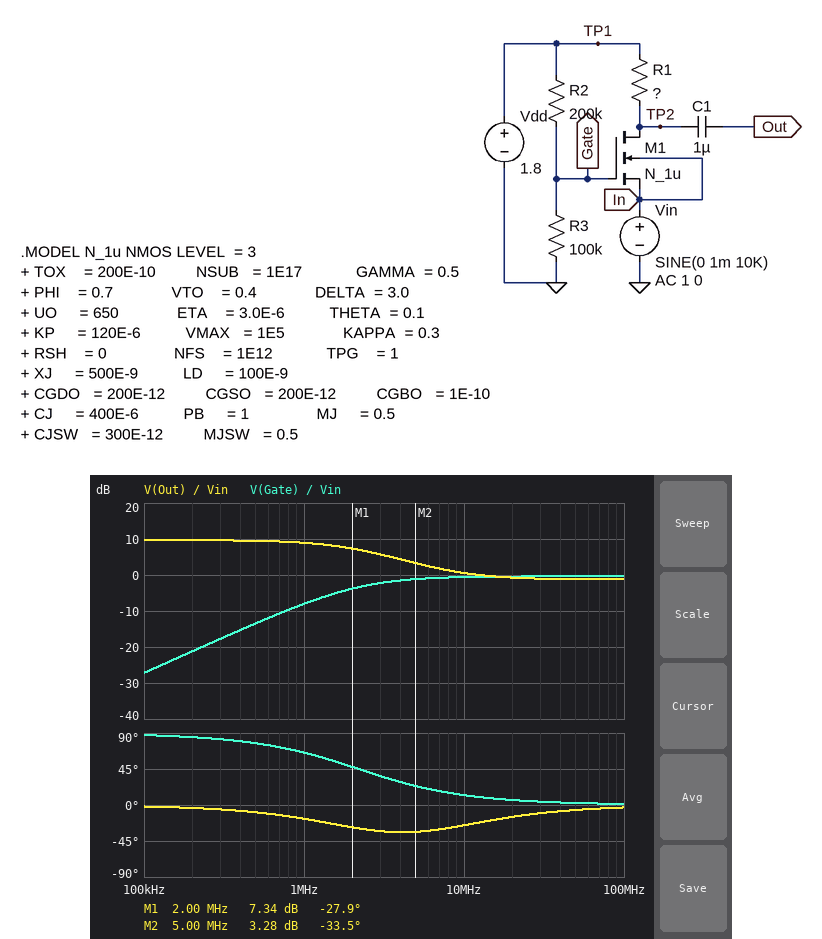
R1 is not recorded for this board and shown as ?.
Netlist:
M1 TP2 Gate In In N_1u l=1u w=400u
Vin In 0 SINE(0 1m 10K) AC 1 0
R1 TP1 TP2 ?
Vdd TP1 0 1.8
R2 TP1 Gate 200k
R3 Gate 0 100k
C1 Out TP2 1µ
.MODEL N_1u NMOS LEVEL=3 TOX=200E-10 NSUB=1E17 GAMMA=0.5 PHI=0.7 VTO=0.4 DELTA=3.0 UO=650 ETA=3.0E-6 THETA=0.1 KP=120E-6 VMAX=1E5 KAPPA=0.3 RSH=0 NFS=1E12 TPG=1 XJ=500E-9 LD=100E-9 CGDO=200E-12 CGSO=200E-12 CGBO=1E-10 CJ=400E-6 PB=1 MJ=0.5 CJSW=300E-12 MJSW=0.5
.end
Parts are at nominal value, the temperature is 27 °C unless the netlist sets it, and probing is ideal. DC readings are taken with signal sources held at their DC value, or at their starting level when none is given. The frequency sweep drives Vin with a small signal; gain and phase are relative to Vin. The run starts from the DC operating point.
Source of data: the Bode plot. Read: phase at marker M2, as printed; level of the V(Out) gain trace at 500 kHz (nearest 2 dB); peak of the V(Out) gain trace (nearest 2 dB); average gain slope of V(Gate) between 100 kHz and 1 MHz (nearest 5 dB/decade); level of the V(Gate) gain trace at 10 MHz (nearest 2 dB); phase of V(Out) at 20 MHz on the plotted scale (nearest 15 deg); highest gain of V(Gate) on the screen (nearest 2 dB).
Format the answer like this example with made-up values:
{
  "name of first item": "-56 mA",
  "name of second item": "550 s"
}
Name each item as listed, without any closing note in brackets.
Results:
{
  "phase at marker M2, as printed": "-33.5 deg",
  "level of the V(Out) gain trace at 500 kHz": "10 dB",
  "peak of the V(Out) gain trace": "10 dB",
  "average gain slope of V(Gate) between 100 kHz and 1 MHz": "20 dB/decade",
  "level of the V(Gate) gain trace at 10 MHz": "0 dB",
  "phase of V(Out) at 20 MHz on the plotted scale": "-15 deg",
  "highest gain of V(Gate) on the screen": "0 dB"
}
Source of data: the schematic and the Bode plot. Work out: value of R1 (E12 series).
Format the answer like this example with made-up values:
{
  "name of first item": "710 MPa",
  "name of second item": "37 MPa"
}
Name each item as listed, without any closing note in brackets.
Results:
{
  "value of R1": "1.2 kΩ"
}
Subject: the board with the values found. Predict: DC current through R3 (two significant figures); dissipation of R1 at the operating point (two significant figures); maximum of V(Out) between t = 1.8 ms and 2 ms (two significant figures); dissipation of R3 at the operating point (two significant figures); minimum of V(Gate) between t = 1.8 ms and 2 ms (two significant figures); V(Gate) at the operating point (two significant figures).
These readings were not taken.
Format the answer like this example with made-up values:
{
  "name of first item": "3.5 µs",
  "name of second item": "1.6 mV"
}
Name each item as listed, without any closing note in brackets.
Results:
{
  "DC current through R3": "6.0 µA",
  "dissipation of R1 at the operating point": "2.2 mW",
  "maximum of V(Out) between t = 1.8 ms and 2 ms": "3.1 mV",
  "dissipation of R3 at the operating point": "3.6 µW",
  "minimum of V(Gate) between t = 1.8 ms and 2 ms": "600 mV",
  "V(Gate) at the operating point": "600 mV"
}
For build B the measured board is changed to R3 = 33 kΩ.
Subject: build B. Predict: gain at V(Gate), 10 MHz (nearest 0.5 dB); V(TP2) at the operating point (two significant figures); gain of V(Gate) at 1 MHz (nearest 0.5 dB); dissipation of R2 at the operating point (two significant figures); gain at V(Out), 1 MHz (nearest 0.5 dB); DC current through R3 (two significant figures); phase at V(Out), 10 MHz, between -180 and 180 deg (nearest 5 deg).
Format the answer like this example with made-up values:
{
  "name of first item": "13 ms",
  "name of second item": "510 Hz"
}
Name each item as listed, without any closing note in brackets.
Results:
{
  "gain at V(Gate), 10 MHz": "-5.0 dB",
  "V(TP2) at the operating point": "1.8 V",
  "gain of V(Gate) at 1 MHz": "-22.5 dB",
  "dissipation of R2 at the operating point": "12 µW",
  "gain at V(Out), 1 MHz": "-17.5 dB",
  "DC current through R3": "7.7 µA",
  "phase at V(Out), 10 MHz, between -180 and 180 deg": "-35 deg"
}
